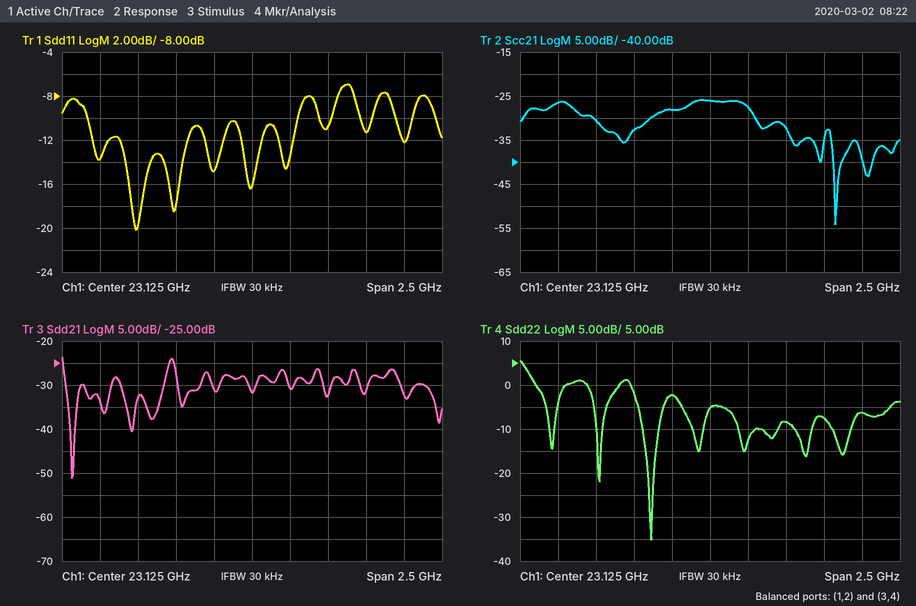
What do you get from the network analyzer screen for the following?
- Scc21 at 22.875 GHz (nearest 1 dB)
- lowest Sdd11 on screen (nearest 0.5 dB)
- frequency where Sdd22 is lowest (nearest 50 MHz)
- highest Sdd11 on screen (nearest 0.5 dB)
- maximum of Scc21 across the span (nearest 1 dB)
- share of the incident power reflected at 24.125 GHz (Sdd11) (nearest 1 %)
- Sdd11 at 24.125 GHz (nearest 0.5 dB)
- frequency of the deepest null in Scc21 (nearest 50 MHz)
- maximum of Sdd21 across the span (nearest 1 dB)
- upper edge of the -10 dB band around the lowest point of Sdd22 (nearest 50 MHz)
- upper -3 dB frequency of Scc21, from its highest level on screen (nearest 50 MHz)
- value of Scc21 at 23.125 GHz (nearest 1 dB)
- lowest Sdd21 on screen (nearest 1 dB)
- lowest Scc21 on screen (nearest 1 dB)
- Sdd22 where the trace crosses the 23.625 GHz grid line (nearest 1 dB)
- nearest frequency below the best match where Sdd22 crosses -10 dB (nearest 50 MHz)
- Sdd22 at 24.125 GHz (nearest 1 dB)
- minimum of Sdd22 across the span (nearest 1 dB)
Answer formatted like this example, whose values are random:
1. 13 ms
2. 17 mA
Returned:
1. -28 dB
2. -20.0 dB
3. 22.75 GHz
4. -7.0 dB
5. -26 dB
6. 6 %
7. -12.0 dB
8. 23.95 GHz
9. -24 dB
10. 22.80 GHz
11. 23.40 GHz
12. -26 dB
13. -51 dB
14. -54 dB
15. -8 dB
16. 22.70 GHz
17. -6 dB
18. -35 dB
